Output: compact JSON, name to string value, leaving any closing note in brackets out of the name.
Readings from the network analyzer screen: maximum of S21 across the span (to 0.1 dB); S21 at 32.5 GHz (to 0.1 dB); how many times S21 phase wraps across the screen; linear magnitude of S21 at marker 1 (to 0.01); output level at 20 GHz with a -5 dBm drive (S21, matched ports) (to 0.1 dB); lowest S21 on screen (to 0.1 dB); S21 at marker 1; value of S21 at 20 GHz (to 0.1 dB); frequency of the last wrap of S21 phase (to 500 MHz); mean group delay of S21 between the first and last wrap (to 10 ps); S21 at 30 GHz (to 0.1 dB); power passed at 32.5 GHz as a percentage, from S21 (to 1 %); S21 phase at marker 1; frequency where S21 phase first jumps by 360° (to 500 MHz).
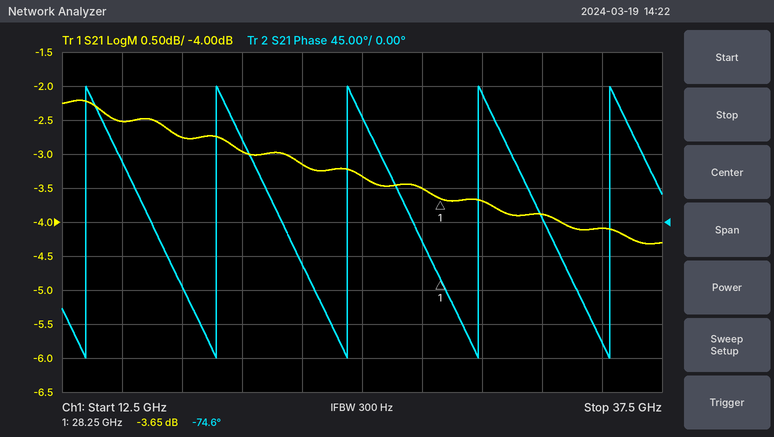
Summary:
{"maximum of S21 across the span": "-2.2 dB", "S21 at 32.5 GHz": "-3.9 dB", "how many times S21 phase wraps across the screen": "5", "linear magnitude of S21 at marker 1": "0.66", "output level at 20 GHz with a -5 dBm drive (S21, matched ports)": "-8.0 dBm", "lowest S21 on screen": "-4.3 dB", "S21 at marker 1": "-3.65 dB", "value of S21 at 20 GHz": "-3.0 dB", "frequency of the last wrap of S21 phase": "35.5 GHz", "mean group delay of S21 between the first and last wrap": "180 ps", "S21 at 30 GHz": "-3.7 dB", "power passed at 32.5 GHz as a percentage, from S21": "41 %", "S21 phase at marker 1": "-74.6°", "frequency where S21 phase first jumps by 360°": "13.5 GHz"}
